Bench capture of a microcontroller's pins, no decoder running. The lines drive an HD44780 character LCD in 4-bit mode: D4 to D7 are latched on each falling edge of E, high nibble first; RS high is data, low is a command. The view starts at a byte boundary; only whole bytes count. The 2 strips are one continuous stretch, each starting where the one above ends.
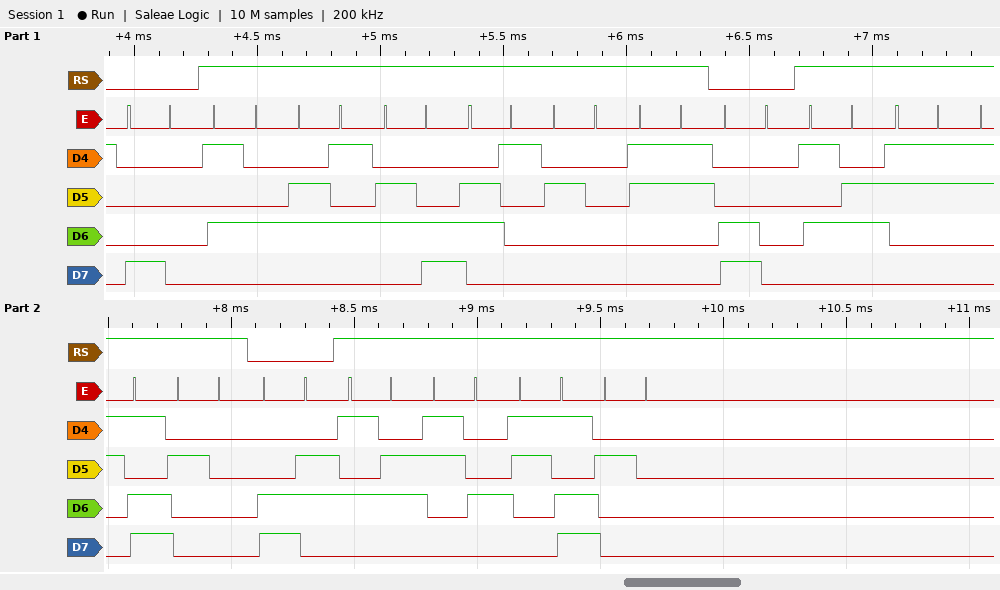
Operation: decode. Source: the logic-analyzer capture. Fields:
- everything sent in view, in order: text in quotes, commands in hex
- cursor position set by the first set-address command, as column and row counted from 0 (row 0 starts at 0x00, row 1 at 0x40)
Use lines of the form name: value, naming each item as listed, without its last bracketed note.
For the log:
everything sent in view, in order: text in quotes, commands in hex: 0x80 "Tela 3" 0xC0 "V3= " 0xC6 "V4= "
cursor position set by the first set-address command, as column and row counted from 0: column 0, row 0
